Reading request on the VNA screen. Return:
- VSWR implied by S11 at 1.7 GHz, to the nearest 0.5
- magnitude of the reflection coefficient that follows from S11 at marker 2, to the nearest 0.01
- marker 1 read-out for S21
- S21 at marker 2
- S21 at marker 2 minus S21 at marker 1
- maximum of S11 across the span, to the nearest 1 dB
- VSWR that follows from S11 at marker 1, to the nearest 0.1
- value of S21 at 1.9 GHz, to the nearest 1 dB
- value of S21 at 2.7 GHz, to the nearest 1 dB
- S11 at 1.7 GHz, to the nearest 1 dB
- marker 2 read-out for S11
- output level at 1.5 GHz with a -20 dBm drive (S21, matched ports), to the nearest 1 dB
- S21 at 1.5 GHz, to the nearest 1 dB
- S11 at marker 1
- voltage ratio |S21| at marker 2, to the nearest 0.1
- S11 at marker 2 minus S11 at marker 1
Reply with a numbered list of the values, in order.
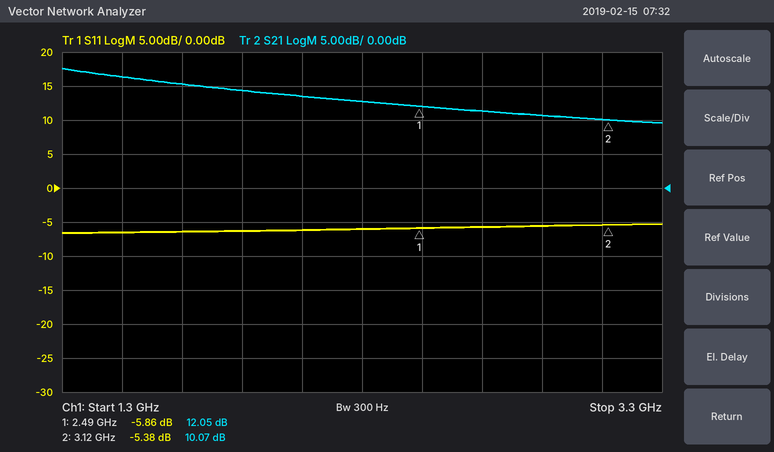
1. 3.0
2. 0.54
3. 12.05 dB
4. 10.07 dB
5. -1.98 dB
6. -5 dB
7. 3.1
8. 14 dB
9. 11 dB
10. -6 dB
11. -5.38 dB
12. -4 dBm
13. 16 dB
14. -5.86 dB
15. 3.2
16. 0.48 dB
